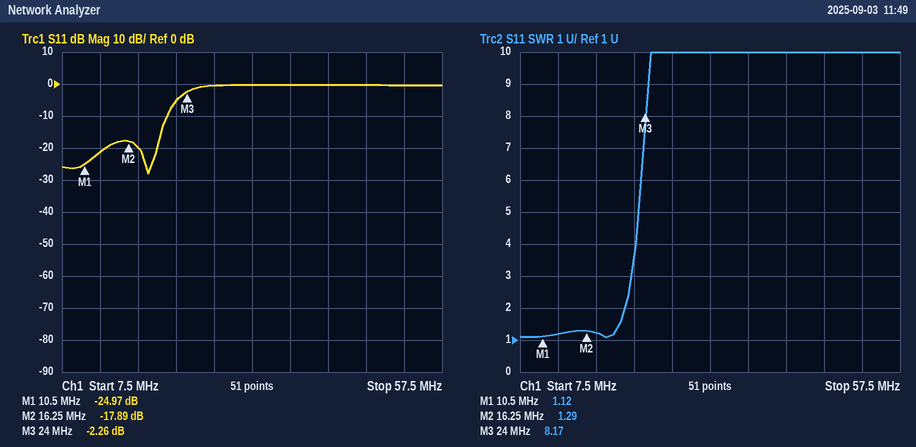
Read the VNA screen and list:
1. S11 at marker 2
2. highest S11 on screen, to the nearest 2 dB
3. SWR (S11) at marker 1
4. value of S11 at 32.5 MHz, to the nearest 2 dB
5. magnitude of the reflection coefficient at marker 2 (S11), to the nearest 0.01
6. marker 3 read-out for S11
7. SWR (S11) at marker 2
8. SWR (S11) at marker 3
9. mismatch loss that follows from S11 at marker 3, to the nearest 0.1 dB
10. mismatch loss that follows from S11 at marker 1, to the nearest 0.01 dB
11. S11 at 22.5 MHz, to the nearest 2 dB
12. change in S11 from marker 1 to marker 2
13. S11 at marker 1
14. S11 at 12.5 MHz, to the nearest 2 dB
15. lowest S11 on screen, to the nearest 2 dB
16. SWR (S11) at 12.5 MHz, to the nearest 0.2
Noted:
-17.89 dB
0 dB
1.12
0 dB
0.13
-2.26 dB
1.29
8.17
3.9 dB
0.01 dB
-6 dB
7.08 dB
-24.97 dB
-22 dB
-28 dB
1.2
